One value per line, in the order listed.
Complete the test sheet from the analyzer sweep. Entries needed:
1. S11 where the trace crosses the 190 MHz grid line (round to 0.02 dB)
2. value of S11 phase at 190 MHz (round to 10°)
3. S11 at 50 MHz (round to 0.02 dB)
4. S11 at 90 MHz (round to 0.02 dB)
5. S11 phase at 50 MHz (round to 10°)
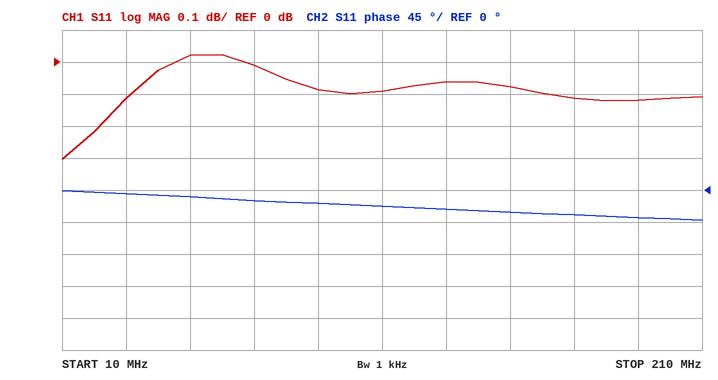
-0.12 dB
-40°
0.02 dB
-0.08 dB
-10°
